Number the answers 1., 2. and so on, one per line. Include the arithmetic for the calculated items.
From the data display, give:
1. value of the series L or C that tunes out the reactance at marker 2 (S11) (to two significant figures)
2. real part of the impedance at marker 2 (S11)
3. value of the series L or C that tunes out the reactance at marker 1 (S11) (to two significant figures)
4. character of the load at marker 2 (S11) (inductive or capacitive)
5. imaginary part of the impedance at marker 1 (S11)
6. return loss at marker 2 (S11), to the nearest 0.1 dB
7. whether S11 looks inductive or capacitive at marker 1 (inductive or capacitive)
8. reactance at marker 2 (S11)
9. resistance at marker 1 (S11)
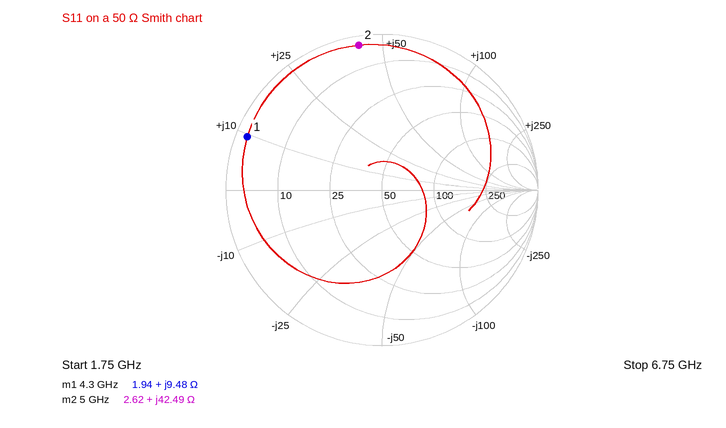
1. C = 1/(2π × 5 GHz × 42.49 Ω) ≈ 749 fF, so 750 fF to two significant figures
2. 2.62 Ω
3. C = 1/(2π × 4.3 GHz × 9.48 Ω) ≈ 3.9 pF
4. inductive
5. +9.48 Ω
6. 0.5 dB
7. inductive
8. +42.49 Ω
9. 1.94 Ω
